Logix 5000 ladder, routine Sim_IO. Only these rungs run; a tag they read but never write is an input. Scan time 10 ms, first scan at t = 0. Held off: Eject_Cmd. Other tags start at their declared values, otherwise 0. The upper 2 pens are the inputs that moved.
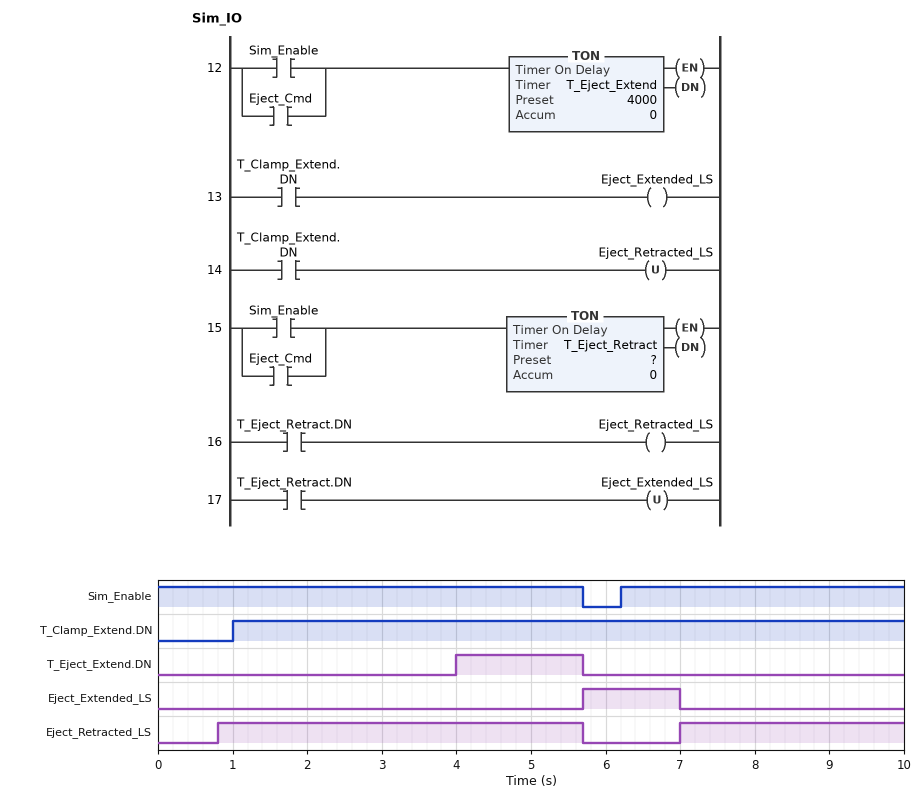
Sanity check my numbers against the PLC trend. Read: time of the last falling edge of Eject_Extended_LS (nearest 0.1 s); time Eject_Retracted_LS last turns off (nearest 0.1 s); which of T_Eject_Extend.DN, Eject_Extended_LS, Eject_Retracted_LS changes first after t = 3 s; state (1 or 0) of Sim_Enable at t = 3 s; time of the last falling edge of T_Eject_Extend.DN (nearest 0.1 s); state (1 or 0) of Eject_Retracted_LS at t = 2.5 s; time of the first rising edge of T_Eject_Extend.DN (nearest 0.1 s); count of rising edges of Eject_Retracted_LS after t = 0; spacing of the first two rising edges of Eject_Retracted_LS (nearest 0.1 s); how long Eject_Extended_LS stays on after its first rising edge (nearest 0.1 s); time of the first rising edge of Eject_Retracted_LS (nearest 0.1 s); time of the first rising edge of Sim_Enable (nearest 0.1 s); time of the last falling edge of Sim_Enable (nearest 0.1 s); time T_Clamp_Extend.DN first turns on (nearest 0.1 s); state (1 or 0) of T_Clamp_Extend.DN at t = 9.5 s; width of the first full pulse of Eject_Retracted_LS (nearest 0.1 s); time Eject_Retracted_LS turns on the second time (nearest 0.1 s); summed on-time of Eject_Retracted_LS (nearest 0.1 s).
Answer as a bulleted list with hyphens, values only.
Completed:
- 7.0 s
- 5.7 s
- T_Eject_Extend.DN
- 1
- 5.7 s
- 1
- 4.0 s
- 2
- 6.2 s
- 1.3 s
- 0.8 s
- 6.2 s
- 5.7 s
- 1.0 s
- 1
- 4.9 s
- 7.0 s
- 7.9 s
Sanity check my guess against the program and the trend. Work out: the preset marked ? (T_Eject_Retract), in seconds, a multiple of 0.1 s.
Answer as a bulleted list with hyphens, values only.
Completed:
- 0.8 s
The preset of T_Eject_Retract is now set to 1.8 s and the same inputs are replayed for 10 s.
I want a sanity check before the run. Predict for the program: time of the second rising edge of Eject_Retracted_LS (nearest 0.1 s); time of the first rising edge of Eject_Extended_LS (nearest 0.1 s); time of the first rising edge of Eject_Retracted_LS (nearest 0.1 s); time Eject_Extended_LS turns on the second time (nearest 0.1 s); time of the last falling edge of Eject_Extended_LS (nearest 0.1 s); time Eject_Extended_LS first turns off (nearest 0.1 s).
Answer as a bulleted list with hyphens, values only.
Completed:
- 8.0 s
- 1.0 s
- 1.8 s
- 5.7 s
- 8.0 s
- 1.8 s
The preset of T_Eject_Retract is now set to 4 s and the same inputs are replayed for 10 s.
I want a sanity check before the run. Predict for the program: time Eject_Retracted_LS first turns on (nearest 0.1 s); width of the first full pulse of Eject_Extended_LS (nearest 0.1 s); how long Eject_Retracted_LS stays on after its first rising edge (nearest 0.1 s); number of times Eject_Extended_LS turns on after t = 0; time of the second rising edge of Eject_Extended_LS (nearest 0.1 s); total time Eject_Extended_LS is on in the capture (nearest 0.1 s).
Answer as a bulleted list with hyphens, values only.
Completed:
- 4.0 s
- 3.0 s
- 1.7 s
- 2
- 5.7 s
- 7.3 s
